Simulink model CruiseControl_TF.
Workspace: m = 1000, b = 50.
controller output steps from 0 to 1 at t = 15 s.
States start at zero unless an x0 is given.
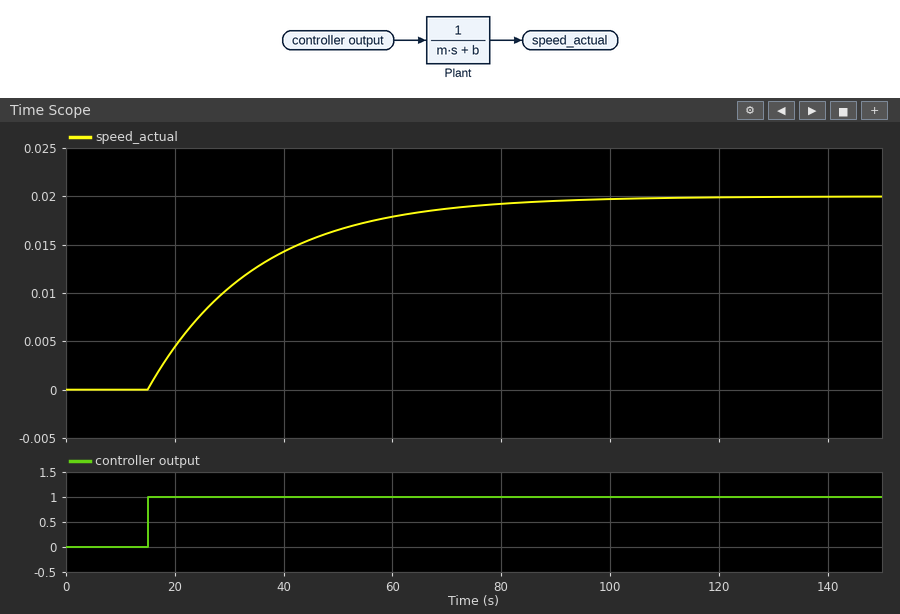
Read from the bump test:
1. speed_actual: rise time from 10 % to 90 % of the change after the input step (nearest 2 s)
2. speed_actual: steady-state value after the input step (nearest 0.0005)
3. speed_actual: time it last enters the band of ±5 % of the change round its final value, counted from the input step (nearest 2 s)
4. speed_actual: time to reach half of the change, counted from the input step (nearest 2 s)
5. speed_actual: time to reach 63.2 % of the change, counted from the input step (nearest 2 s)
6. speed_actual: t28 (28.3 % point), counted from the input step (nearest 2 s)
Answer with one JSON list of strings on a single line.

["44 s", "0.0200", "60 s", "14 s", "20 s", "6 s"]
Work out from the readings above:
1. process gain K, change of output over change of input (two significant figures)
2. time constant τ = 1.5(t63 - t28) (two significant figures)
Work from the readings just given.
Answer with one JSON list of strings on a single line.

["0.020", "21 s"]
